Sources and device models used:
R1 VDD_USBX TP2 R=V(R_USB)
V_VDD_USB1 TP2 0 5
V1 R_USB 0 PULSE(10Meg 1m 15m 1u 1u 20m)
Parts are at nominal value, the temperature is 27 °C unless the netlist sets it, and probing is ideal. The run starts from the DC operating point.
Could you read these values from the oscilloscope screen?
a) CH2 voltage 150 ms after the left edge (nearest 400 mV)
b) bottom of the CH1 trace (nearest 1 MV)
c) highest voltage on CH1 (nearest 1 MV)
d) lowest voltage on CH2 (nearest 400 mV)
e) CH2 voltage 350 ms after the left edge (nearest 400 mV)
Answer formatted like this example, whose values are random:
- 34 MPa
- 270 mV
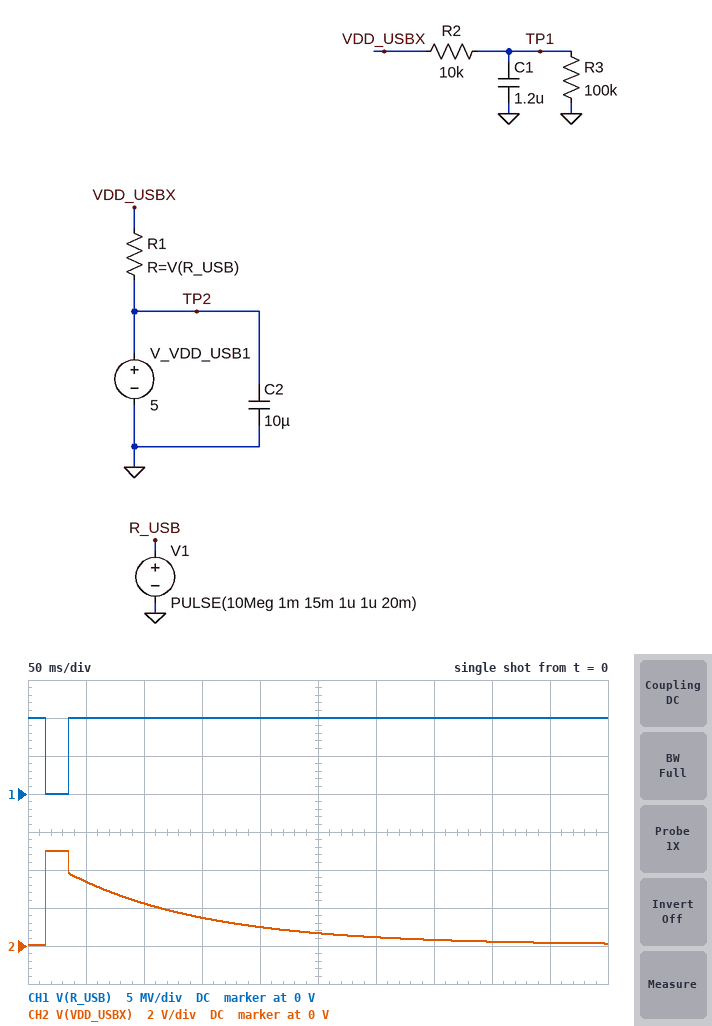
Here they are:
- 1.6 V
- 0 V
- 10 MV
- 0 V
- 400 mV
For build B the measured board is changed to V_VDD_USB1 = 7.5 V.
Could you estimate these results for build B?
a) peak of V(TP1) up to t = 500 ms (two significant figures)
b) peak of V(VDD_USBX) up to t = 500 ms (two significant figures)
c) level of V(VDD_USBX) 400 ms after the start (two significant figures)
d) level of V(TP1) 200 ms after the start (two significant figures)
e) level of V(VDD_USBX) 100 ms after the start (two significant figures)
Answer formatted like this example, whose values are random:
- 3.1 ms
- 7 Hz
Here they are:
- 5.7 V
- 7.5 V
- 340 mV
- 1.5 V
- 3.4 V
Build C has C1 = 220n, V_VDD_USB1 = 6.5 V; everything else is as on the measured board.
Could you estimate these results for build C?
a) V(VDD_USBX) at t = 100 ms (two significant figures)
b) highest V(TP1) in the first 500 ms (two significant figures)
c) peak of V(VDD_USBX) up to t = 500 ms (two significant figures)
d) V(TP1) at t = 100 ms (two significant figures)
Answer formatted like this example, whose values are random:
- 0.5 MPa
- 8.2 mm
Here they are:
- 370 mV
- 5.9 V
- 6.5 V
- 360 mV
